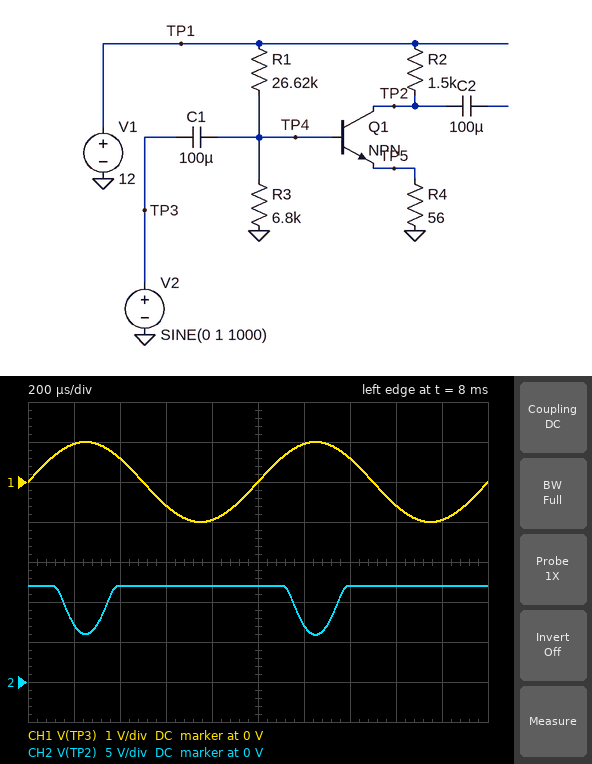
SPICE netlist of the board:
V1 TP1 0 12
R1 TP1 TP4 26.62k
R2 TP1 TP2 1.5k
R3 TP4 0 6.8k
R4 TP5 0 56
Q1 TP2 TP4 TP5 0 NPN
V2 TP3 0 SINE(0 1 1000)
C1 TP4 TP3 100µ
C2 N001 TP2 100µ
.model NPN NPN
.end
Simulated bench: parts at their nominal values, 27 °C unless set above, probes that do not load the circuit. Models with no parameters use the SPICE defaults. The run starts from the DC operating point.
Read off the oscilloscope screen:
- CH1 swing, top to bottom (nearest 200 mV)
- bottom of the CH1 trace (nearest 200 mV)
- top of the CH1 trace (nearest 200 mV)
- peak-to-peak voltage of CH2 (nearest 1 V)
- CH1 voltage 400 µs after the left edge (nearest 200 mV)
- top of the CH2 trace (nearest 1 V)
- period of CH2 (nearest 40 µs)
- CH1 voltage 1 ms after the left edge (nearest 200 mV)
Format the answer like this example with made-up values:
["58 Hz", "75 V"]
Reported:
["2.0 V", "-1.0 V", "1.0 V", "6 V", "600 mV", "12 V", "1.00 ms", "0 V"]
